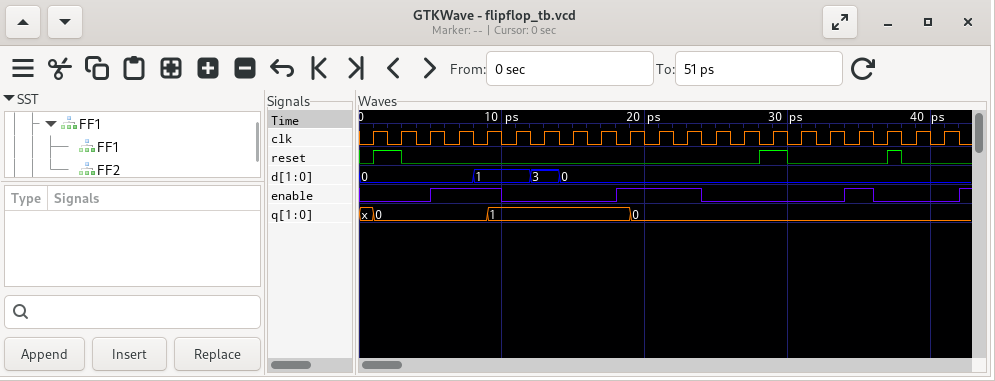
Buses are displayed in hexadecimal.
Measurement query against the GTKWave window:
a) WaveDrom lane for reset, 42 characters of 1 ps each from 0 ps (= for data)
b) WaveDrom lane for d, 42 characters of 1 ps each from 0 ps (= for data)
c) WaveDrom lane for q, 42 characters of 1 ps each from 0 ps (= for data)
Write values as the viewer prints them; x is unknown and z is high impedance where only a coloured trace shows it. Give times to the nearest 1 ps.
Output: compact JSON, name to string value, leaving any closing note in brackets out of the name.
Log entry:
{"WaveDrom lane for reset, 42 characters of 1 ps each from 0 ps": "{name: 'reset', wave: '01.0........................1.0......10...'}", "WaveDrom lane for d, 42 characters of 1 ps each from 0 ps": "{name: 'd', wave: '=.......=...=.=...........................', data: '0 1 3 0'}", "WaveDrom lane for q, 42 characters of 1 ps each from 0 ps": "{name: 'q', wave: 'x=.......=.........=......................', data: '0 1 0'}"}
